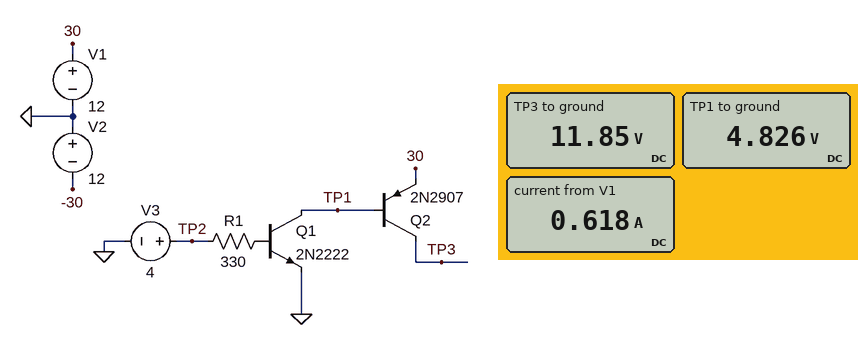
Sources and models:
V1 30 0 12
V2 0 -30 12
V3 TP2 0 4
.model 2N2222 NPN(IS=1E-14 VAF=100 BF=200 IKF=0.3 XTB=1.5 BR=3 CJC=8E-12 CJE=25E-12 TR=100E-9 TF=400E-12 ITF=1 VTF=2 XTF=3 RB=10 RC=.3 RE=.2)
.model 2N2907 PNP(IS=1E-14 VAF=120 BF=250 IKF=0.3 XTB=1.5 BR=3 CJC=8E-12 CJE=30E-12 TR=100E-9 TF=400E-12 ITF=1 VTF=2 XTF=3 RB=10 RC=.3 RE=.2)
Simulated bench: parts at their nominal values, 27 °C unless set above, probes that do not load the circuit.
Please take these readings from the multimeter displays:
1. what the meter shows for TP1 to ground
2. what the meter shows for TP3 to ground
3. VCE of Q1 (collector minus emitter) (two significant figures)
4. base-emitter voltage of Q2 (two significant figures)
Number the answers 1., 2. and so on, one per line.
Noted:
1. 4.826 V
2. 11.85 V
3. 4.8 V
4. -7.2 V
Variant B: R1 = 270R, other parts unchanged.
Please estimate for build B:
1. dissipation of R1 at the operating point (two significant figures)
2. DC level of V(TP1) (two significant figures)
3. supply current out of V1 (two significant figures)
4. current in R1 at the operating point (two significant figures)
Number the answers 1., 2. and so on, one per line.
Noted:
1. 31 mW
2. 4.1 V
3. 690 mA
4. 11 mA
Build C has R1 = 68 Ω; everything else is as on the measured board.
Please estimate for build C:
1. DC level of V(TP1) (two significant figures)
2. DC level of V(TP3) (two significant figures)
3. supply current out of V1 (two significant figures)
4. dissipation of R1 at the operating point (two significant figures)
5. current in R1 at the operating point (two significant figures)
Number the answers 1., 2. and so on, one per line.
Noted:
1. 640 mV
2. 12 V
3. 1.0 A
4. 95 mW
5. 37 mA
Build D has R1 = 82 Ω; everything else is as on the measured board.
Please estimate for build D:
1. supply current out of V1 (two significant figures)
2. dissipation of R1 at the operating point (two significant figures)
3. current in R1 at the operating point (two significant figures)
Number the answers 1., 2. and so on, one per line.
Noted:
1. 1.0 A
2. 82 mW
3. 32 mA
